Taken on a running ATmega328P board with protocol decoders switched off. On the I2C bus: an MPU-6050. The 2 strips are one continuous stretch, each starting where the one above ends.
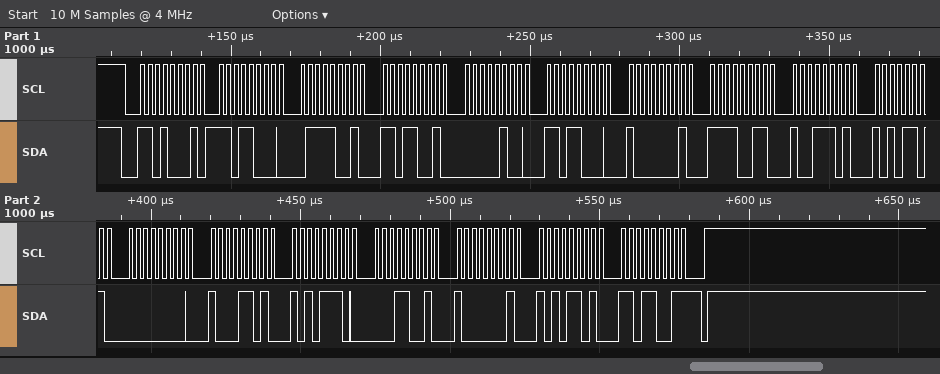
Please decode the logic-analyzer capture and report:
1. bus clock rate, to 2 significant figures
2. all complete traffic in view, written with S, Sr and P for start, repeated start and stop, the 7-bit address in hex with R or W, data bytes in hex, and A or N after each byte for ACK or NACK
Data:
400 kHz
S 68R A D8 A 79 A D9 A 04 A D8 A 81 A F3 A 9D A AD A 00 A 8D A AE A 19 A 81 A AD A D9 N P
